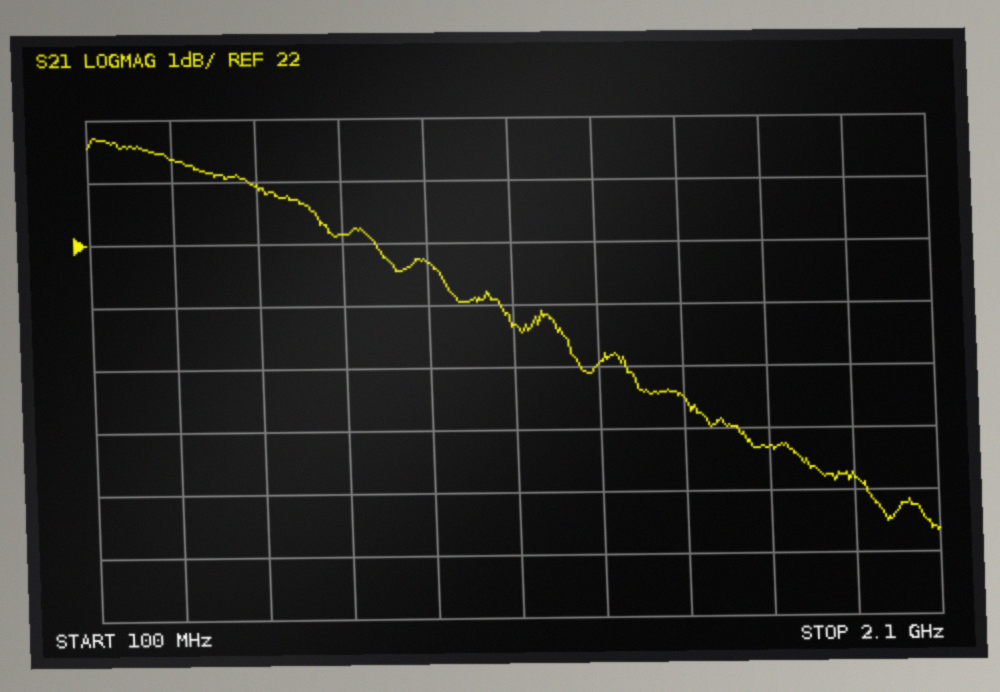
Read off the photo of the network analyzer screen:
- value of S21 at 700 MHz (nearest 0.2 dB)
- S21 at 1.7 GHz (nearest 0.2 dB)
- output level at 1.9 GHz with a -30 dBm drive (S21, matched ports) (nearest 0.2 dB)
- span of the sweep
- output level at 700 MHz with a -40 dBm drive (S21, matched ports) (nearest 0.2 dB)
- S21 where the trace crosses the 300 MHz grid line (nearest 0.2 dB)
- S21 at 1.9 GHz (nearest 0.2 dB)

22.2 dB
18.8 dB
-11.8 dBm
2 GHz
-17.8 dBm
23.4 dB
18.2 dB
